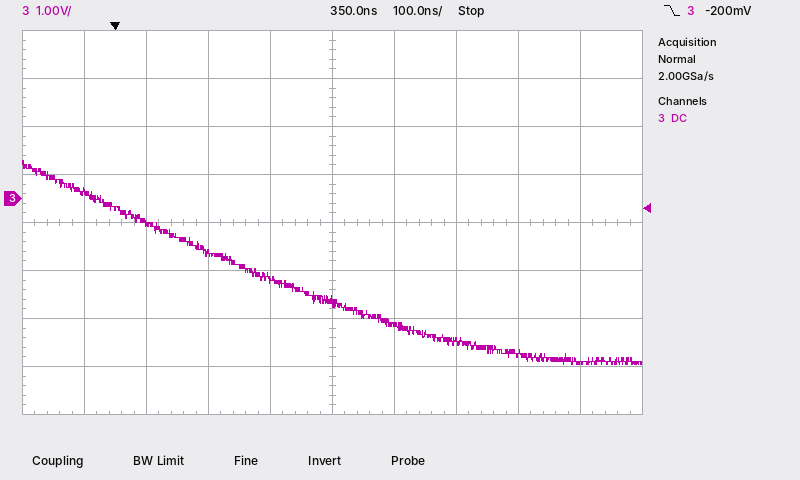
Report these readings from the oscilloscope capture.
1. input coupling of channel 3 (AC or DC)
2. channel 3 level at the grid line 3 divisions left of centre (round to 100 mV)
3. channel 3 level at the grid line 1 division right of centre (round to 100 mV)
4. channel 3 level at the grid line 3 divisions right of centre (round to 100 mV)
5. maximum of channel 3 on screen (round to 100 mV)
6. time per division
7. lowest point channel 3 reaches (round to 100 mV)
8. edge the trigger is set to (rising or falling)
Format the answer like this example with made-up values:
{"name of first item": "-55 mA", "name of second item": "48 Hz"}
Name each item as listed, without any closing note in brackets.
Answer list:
{"input coupling of channel 3": "DC", "channel 3 level at the grid line 3 divisions left of centre": "-500 mV", "channel 3 level at the grid line 1 division right of centre": "-2.6 V", "channel 3 level at the grid line 3 divisions right of centre": "-3.2 V", "maximum of channel 3 on screen": "800 mV", "time per division": "100 ns", "lowest point channel 3 reaches": "-3.5 V", "edge the trigger is set to": "falling"}
